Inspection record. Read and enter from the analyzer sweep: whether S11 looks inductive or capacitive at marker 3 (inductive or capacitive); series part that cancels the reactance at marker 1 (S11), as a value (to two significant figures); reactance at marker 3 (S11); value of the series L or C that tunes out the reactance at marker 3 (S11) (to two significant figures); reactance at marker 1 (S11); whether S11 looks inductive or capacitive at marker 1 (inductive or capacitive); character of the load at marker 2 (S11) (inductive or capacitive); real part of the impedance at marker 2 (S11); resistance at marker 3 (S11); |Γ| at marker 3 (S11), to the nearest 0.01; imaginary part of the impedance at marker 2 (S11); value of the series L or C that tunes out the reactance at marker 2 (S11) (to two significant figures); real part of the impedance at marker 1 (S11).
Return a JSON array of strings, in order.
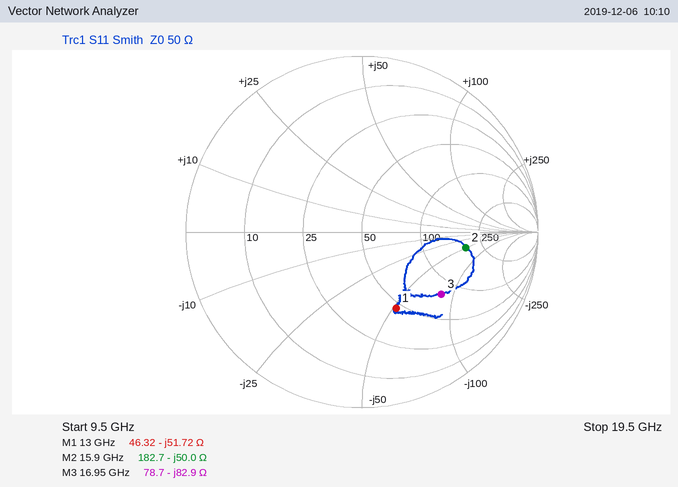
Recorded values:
["capacitive", "630 pH", "-82.9 Ω", "780 pH", "-51.72 Ω", "capacitive", "capacitive", "182.7 Ω", "78.7 Ω", "0.57", "-50.0 Ω", "500 pH", "46.32 Ω"]
